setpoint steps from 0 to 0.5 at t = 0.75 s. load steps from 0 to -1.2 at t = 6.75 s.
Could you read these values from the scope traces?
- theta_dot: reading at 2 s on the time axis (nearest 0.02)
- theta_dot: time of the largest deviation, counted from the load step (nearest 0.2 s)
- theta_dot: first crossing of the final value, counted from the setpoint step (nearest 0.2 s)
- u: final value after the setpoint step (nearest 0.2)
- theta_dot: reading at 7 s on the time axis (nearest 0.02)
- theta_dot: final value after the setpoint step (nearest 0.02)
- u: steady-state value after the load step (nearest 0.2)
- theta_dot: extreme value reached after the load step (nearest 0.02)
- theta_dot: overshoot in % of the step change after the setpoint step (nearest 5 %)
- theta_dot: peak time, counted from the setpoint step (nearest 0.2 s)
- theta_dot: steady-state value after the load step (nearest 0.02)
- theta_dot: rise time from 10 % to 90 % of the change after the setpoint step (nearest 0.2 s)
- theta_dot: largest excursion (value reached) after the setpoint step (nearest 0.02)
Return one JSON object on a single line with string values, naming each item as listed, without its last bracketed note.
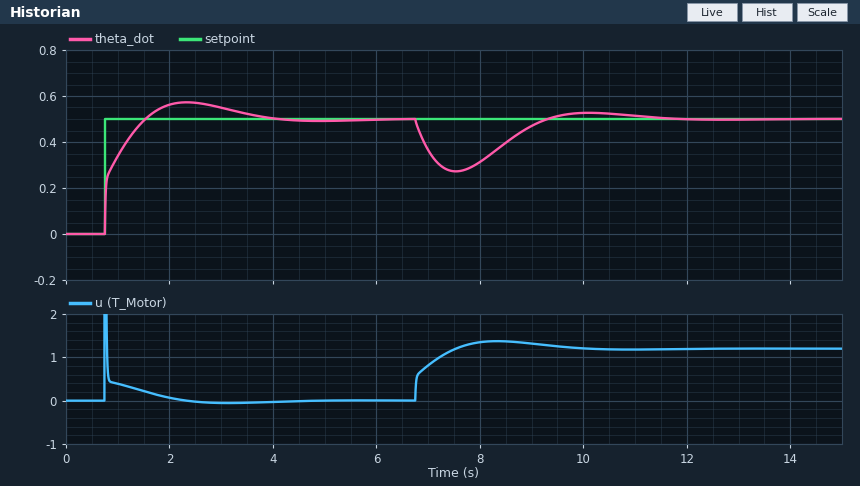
{"theta_dot: reading at 2 s on the time axis": "0.56", "theta_dot: time of the largest deviation, counted from the load step": "0.8 s", "theta_dot: first crossing of the final value, counted from the setpoint step": "0.8 s", "u: final value after the setpoint step": "0.0", "theta_dot: reading at 7 s on the time axis": "0.36", "theta_dot: final value after the setpoint step": "0.50", "u: steady-state value after the load step": "1.2", "theta_dot: extreme value reached after the load step": "0.28", "theta_dot: overshoot in % of the step change after the setpoint step": "15 %", "theta_dot: peak time, counted from the setpoint step": "1.6 s", "theta_dot: steady-state value after the load step": "0.50", "theta_dot: rise time from 10 % to 90 % of the change after the setpoint step": "0.6 s", "theta_dot: largest excursion (value reached) after the setpoint step": "0.58"}
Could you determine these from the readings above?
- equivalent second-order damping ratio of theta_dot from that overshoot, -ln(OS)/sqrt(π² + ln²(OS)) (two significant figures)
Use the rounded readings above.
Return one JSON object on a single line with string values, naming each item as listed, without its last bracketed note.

{"equivalent second-order damping ratio of theta_dot from that overshoot, -ln(OS)/sqrt(π² + ln²(OS))": "0.52"}
